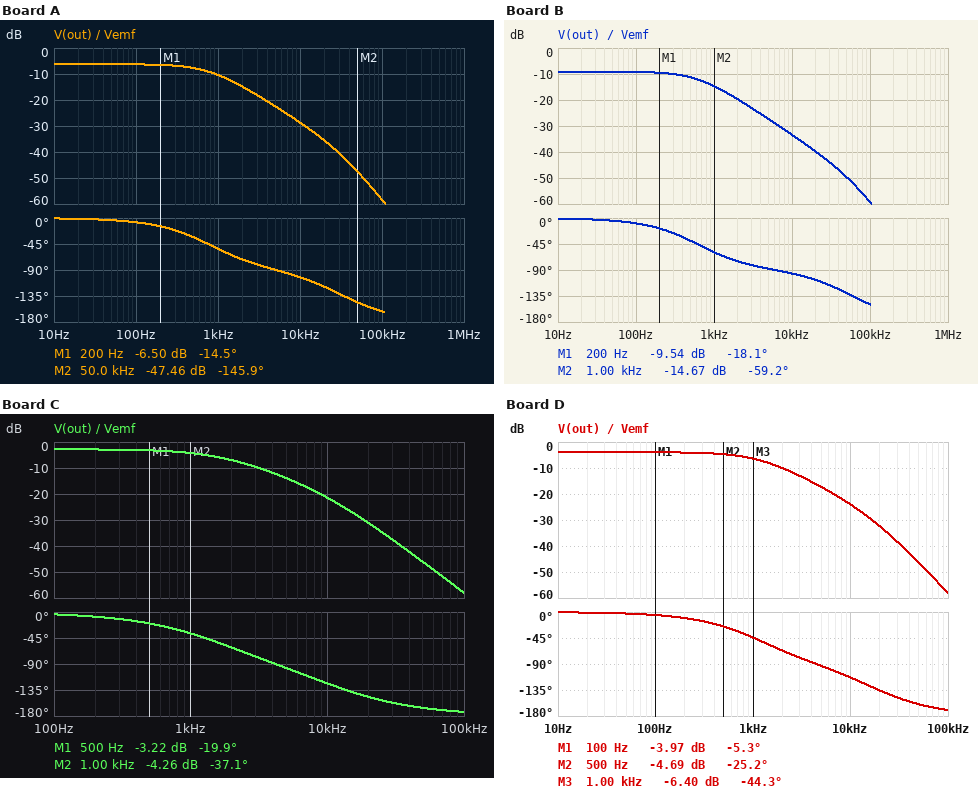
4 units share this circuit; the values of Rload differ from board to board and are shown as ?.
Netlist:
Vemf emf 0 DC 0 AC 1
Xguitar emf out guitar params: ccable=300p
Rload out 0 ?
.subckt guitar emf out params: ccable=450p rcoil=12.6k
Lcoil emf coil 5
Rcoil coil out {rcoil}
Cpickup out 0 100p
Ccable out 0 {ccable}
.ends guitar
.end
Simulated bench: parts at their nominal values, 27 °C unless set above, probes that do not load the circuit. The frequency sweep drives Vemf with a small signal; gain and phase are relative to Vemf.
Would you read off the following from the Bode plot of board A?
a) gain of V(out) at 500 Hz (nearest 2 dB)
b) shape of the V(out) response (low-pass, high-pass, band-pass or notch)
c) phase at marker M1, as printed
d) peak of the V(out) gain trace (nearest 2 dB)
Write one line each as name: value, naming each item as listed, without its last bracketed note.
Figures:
gain of V(out) at 500 Hz: -8 dB
shape of the V(out) response: low-pass
phase at marker M1, as printed: -14.5 deg
peak of the V(out) gain trace: -6 dB
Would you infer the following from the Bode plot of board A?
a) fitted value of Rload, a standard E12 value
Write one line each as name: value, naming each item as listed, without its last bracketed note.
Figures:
fitted value of Rload, a standard E12 value: 12 kΩ
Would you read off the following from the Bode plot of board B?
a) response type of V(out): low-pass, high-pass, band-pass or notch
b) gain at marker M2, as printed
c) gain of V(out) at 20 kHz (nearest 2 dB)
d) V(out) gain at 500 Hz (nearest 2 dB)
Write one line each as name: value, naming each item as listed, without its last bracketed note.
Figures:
response type of V(out): low-pass, high-pass, band-pass or notch: low-pass
gain at marker M2, as printed: -14.67 dB
gain of V(out) at 20 kHz: -40 dB
V(out) gain at 500 Hz: -12 dB
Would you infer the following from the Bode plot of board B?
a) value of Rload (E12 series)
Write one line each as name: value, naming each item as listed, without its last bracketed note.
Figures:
value of Rload: 6.8 kΩ
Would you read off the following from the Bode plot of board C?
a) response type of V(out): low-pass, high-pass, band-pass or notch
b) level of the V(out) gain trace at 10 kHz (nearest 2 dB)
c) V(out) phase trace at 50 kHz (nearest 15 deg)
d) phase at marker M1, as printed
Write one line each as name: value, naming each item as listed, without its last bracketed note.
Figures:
response type of V(out): low-pass, high-pass, band-pass or notch: low-pass
level of the V(out) gain trace at 10 kHz: -22 dB
V(out) phase trace at 50 kHz: -165 deg
phase at marker M1, as printed: -19.9 deg
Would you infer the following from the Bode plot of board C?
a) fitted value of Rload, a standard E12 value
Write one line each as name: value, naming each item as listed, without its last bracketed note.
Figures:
fitted value of Rload, a standard E12 value: 33 kΩ
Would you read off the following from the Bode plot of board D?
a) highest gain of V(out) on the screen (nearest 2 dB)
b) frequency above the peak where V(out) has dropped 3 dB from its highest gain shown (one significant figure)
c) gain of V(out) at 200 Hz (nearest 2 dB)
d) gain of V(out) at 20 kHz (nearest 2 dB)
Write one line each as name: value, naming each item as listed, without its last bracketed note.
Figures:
highest gain of V(out) on the screen: -4 dB
frequency above the peak where V(out) has dropped 3 dB from its highest gain shown: 1 kHz
gain of V(out) at 200 Hz: -4 dB
gain of V(out) at 20 kHz: -32 dB
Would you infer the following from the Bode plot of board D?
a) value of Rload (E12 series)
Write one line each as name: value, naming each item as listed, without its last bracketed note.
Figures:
value of Rload: 22 kΩ
